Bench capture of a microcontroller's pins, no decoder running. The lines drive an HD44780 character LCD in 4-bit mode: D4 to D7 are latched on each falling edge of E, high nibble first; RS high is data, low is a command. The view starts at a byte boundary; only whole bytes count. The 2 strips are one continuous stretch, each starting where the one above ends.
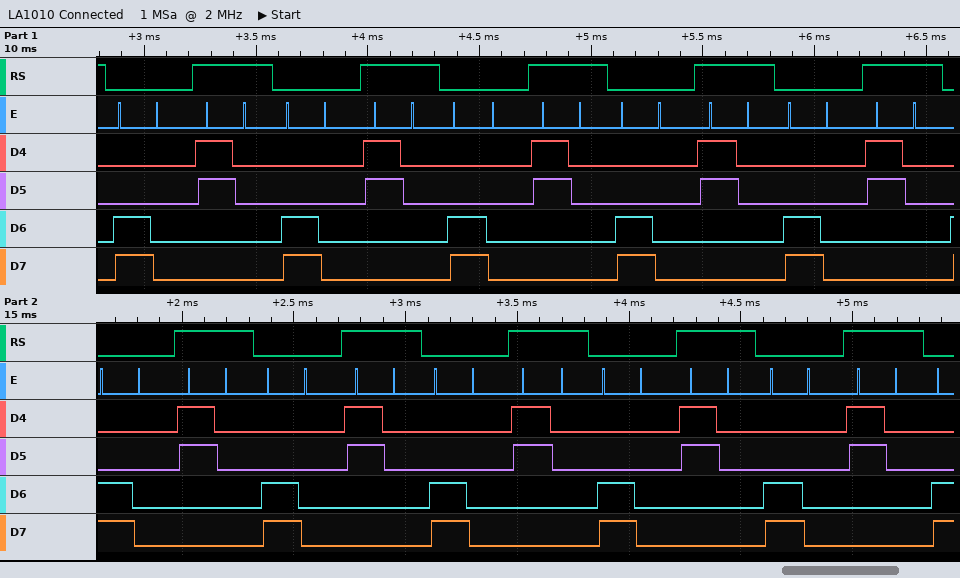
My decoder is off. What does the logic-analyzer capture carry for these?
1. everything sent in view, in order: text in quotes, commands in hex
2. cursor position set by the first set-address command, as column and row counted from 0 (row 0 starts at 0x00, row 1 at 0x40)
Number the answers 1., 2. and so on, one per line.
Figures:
1. 0xC0 "0" 0xC0 "0" 0xC0 "0" 0xC0 "0" 0xC0 "0" 0xC0 "0" 0xC0 "0" 0xC0 "0" 0xC0 "0" 0xC0 "0"
2. column 0, row 1
